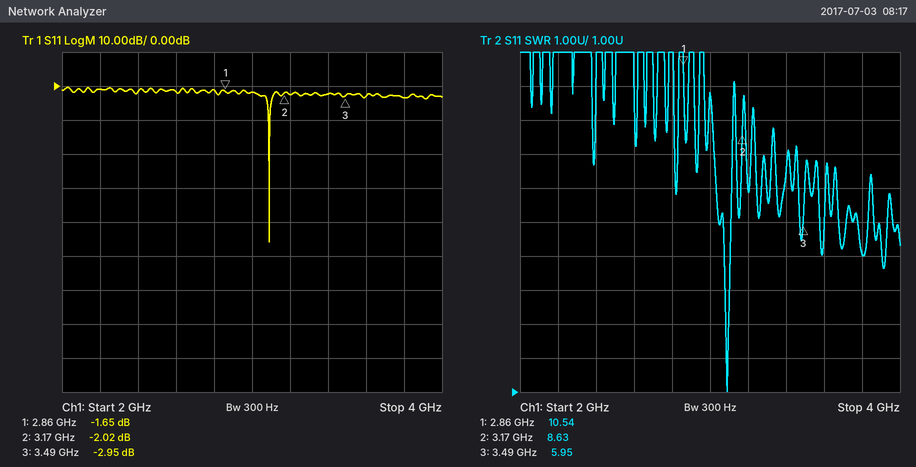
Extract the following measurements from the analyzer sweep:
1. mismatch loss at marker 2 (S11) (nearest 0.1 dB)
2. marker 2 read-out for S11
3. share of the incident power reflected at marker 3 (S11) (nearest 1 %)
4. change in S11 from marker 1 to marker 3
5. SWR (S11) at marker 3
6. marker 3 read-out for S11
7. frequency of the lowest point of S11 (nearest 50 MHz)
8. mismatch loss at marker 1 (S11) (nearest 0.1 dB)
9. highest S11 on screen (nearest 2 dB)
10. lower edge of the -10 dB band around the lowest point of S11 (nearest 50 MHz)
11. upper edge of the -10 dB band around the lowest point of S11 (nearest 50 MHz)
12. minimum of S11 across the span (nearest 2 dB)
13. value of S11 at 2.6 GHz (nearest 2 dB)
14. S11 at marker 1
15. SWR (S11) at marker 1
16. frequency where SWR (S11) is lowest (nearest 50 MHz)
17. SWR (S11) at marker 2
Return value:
4.3 dB
-2.02 dB
51 %
-1.30 dB
5.95
-2.95 dB
3.10 GHz
5.0 dB
0 dB
3.10 GHz
3.10 GHz
-46 dB
-2 dB
-1.65 dB
10.54
3.10 GHz
8.63
